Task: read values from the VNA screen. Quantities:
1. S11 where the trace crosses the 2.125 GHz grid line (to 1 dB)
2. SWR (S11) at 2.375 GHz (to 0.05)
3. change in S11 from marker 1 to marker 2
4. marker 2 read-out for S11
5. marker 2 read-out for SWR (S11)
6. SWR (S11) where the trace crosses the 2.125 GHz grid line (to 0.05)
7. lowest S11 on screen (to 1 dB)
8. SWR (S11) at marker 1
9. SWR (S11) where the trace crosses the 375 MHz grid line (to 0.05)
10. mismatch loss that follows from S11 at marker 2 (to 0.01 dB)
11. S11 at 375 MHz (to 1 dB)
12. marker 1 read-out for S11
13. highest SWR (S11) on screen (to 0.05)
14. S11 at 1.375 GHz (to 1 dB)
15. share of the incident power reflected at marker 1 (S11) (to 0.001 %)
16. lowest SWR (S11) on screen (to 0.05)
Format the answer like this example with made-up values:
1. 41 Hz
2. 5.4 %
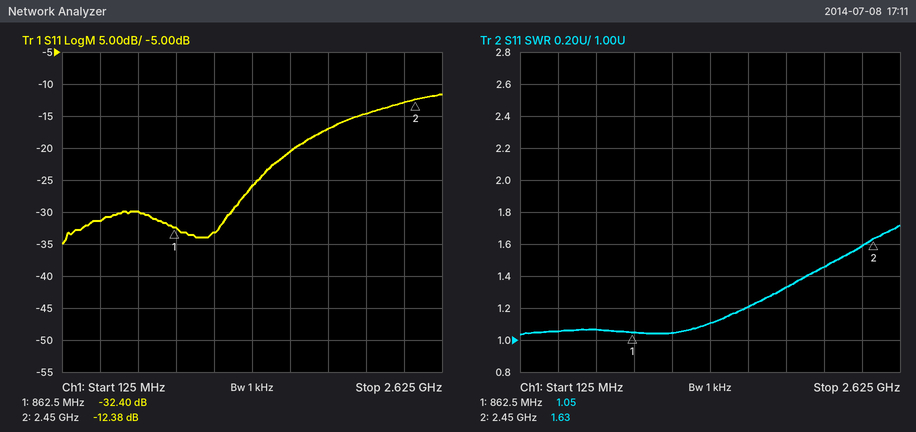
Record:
1. -15 dB
2. 1.60
3. 20.02 dB
4. -12.38 dB
5. 1.63
6. 1.45
7. -35 dB
8. 1.05
9. 1.05
10. 0.26 dB
11. -31 dB
12. -32.40 dB
13. 1.70
14. -26 dB
15. 0.058 %
16. 1.05
